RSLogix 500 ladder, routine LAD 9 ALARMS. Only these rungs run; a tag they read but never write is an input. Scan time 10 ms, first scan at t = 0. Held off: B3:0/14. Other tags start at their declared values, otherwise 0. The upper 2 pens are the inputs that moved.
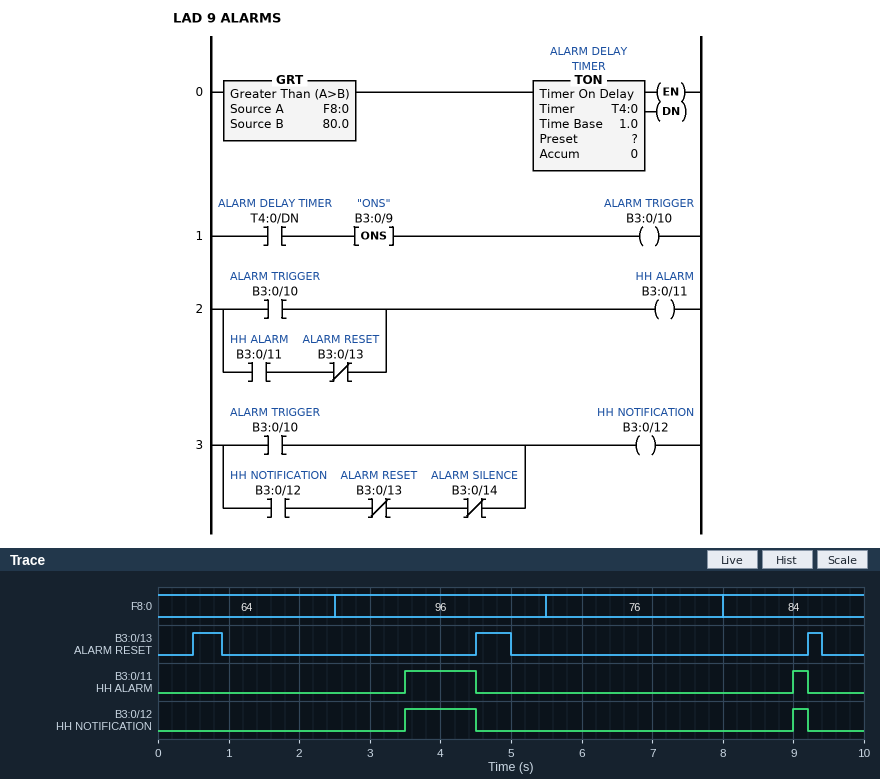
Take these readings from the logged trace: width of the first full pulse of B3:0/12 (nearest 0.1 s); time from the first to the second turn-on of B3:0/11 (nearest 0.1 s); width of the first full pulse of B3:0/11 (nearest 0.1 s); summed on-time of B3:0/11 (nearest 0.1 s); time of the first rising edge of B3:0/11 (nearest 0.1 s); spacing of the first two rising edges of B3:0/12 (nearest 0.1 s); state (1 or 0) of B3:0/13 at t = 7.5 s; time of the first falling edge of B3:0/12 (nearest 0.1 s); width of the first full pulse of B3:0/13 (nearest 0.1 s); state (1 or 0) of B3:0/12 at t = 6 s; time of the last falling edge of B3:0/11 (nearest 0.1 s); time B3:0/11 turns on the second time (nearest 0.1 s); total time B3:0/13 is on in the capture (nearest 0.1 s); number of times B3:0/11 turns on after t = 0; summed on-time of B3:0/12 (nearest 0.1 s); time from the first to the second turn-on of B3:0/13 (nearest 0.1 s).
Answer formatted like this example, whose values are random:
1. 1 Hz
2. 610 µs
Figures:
1. 1.0 s
2. 5.5 s
3. 1.0 s
4. 1.2 s
5. 3.5 s
6. 5.5 s
7. 0
8. 4.5 s
9. 0.4 s
10. 0
11. 9.2 s
12. 9.0 s
13. 1.1 s
14. 2
15. 1.2 s
16. 4.0 s
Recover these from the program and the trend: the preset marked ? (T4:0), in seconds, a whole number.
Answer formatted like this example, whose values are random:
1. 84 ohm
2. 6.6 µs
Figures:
1. 1 s
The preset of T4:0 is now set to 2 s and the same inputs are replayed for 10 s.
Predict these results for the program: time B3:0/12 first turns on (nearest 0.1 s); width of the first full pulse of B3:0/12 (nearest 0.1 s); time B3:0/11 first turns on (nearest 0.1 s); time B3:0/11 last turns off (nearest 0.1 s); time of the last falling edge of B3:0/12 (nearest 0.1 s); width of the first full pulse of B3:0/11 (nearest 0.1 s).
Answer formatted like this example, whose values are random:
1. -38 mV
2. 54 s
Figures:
1. 4.5 s
2. 0.0 s
3. 4.5 s
4. 4.5 s
5. 4.5 s
6. 0.0 s
